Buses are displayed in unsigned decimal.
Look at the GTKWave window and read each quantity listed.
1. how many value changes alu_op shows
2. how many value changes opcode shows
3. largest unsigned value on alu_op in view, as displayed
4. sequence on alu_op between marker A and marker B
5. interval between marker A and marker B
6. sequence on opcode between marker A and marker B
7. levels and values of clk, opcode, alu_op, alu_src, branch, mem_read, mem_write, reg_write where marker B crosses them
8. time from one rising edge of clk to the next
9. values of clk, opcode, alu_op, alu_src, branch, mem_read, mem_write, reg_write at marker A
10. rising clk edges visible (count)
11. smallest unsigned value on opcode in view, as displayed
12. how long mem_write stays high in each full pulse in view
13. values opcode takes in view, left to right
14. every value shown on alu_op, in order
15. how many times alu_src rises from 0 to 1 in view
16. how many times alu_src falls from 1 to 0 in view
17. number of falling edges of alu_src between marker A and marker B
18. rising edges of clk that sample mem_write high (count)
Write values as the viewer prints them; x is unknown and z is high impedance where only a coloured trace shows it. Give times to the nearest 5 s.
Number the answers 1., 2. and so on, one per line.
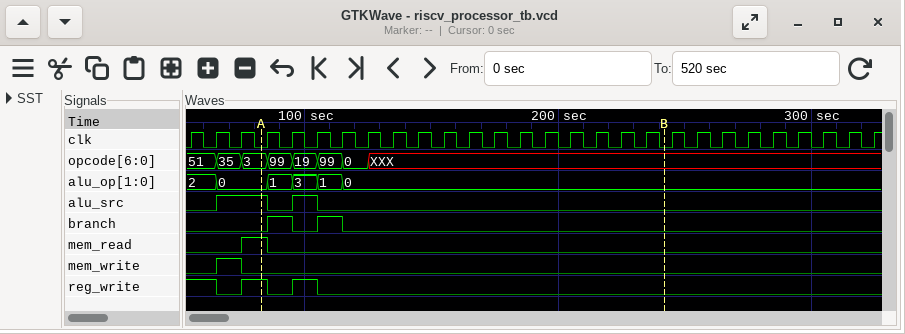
1. 5
2. 7
3. 3
4. 0, 1, 3, 1, 0
5. 160 s
6. 3, 99, 19, 99, 0, XXX
7. clk=0, opcode=XXX, alu_op=0, alu_src=0, branch=0, mem_read=0, mem_write=0, reg_write=0
8. 10 s
9. clk=0, opcode=3, alu_op=0, alu_src=1, branch=0, mem_read=1, mem_write=0, reg_write=1
10. 28
11. 0
12. 10 s
13. 51, 35, 3, 99, 19, 99, 0, XXX
14. 2, 0, 1, 3, 1, 0
15. 2
16. 2
17. 2
18. 1
